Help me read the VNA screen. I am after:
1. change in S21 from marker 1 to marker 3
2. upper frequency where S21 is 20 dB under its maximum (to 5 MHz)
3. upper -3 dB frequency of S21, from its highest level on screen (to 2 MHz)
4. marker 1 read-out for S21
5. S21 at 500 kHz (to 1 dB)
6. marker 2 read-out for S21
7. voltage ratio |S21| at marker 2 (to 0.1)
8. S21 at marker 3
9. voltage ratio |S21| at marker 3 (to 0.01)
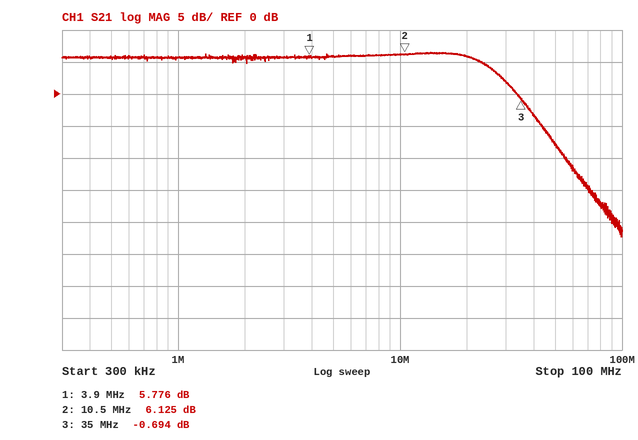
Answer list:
-6.470 dB
65 MHz
26 MHz
5.776 dB
6 dB
6.125 dB
2.0
-0.694 dB
0.92
